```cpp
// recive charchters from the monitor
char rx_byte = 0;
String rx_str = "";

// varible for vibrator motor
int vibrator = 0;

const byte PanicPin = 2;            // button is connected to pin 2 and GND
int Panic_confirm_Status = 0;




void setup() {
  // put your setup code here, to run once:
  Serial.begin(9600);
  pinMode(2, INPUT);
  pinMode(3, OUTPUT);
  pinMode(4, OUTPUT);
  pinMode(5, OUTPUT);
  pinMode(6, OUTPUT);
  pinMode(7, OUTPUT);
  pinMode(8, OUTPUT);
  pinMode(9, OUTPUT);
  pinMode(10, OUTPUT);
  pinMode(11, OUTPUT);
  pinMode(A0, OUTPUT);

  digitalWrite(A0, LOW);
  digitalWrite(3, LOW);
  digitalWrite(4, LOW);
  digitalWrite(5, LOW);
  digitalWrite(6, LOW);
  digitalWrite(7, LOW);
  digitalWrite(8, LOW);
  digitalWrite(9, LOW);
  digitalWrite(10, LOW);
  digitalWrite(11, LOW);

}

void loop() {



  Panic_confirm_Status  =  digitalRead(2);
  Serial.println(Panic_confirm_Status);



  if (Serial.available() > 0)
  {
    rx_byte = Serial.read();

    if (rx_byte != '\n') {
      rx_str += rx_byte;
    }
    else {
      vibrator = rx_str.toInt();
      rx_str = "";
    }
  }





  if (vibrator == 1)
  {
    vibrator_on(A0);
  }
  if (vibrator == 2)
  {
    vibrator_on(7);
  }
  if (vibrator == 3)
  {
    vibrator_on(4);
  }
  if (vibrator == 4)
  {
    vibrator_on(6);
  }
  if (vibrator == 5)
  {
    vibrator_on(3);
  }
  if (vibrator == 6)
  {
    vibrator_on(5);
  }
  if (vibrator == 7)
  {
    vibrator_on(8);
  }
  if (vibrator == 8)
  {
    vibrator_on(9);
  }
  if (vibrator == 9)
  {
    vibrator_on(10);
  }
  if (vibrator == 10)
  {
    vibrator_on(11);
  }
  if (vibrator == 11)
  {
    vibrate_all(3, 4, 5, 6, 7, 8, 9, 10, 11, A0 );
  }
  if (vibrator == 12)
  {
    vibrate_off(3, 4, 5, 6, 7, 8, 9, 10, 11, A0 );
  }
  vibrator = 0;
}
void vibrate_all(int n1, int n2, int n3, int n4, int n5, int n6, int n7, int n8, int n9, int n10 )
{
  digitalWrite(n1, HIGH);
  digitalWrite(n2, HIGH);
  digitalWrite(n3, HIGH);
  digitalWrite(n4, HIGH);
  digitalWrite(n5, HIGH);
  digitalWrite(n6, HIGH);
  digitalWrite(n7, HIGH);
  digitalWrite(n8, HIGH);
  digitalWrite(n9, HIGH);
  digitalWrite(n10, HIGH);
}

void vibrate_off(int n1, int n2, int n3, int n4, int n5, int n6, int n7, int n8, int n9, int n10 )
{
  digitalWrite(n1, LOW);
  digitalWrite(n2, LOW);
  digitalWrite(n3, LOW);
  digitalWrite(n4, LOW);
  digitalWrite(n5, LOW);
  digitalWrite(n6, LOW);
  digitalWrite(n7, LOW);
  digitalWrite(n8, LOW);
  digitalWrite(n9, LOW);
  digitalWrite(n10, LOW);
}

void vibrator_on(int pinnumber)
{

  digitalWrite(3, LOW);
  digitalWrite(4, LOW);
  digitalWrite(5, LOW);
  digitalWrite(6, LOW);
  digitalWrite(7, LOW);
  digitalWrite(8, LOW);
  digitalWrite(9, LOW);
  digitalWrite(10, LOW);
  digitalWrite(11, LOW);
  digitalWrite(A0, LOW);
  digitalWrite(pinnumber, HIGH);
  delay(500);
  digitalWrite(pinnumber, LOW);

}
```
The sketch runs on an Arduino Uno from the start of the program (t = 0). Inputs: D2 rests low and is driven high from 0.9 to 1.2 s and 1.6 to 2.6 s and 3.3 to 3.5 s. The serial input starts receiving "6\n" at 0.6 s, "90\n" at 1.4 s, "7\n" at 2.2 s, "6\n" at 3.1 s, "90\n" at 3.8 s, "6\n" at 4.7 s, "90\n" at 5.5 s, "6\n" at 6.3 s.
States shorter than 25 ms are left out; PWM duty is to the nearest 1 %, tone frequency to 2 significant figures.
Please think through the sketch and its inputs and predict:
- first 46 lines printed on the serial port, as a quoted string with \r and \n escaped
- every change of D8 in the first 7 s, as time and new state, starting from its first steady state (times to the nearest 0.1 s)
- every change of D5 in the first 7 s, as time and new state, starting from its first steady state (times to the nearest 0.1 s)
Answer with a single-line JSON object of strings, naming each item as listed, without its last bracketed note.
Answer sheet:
{"first 46 lines printed on the serial port, as a quoted string with \\r and \\n escaped": "\"0\\r\\n0\\r\\n0\\r\\n0\\r\\n0\\r\\n0\\r\\n0\\r\\n0\\r\\n0\\r\\n0\\r\\n0\\r\\n0\\r\\n0\\r\\n0\\r\\n0\\r\\n0\\r\\n0\\r\\n0\\r\\n0\\r\\n0\\r\\n0\\r\\n0\\r\\n0\\r\\n0\\r\\n0\\r\\n0\\r\\n0\\r\\n0\\r\\n0\\r\\n0\\r\\n0\\r\\n0\\r\\n0\\r\\n0\\r\\n0\\r\\n0\\r\\n0\\r\\n0\\r\\n0\\r\\n0\\r\\n0\\r\\n0\\r\\n0\\r\\n0\\r\\n0\\r\\n0\\r\\n\"", "every change of D8 in the first 7 s, as time and new state, starting from its first steady state": "0 s low; 2.2 s high; 2.7 s low", "every change of D5 in the first 7 s, as time and new state, starting from its first steady state": "0 s low; 0.6 s high; 1.1 s low; 3.1 s high; 3.6 s low; 4.7 s high; 5.2 s low; 6.3 s high; 6.8 s low"}
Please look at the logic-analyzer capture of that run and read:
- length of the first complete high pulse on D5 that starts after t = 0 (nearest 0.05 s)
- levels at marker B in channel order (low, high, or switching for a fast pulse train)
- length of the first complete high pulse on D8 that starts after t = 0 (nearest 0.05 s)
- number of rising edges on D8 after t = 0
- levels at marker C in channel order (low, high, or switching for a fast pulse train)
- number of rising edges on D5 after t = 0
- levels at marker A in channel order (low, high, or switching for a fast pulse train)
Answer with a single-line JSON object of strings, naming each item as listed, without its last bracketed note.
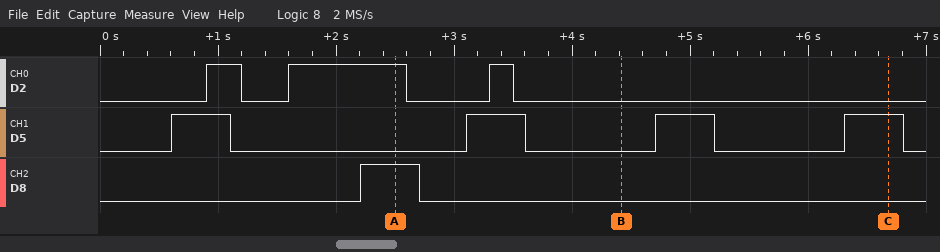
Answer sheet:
{"length of the first complete high pulse on D5 that starts after t = 0": "0.50 s", "levels at marker B in channel order": "D2 low, D5 low, D8 low", "length of the first complete high pulse on D8 that starts after t = 0": "0.50 s", "number of rising edges on D8 after t = 0": "1", "levels at marker C in channel order": "D2 low, D5 high, D8 low", "number of rising edges on D5 after t = 0": "4", "levels at marker A in channel order": "D2 high, D5 low, D8 high"}
